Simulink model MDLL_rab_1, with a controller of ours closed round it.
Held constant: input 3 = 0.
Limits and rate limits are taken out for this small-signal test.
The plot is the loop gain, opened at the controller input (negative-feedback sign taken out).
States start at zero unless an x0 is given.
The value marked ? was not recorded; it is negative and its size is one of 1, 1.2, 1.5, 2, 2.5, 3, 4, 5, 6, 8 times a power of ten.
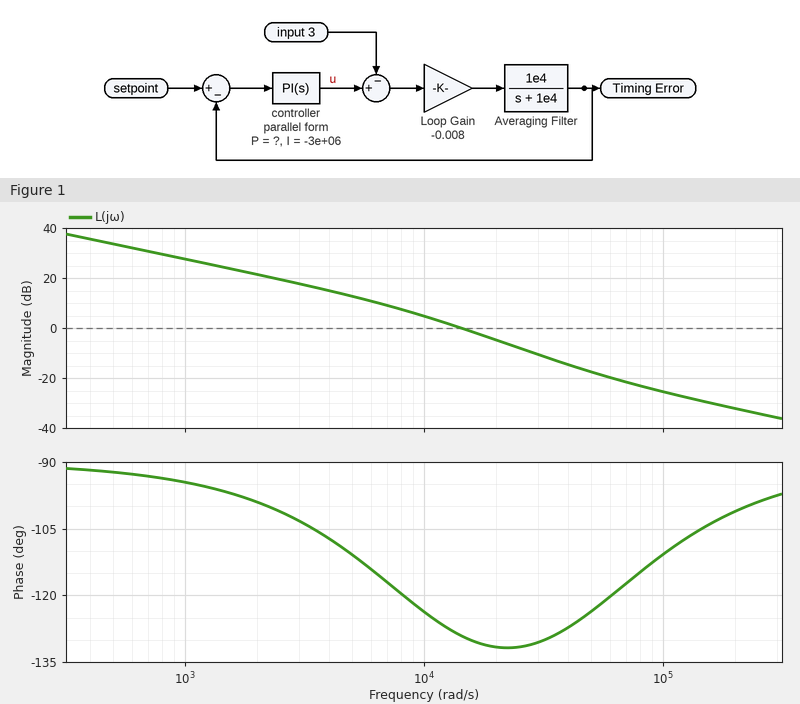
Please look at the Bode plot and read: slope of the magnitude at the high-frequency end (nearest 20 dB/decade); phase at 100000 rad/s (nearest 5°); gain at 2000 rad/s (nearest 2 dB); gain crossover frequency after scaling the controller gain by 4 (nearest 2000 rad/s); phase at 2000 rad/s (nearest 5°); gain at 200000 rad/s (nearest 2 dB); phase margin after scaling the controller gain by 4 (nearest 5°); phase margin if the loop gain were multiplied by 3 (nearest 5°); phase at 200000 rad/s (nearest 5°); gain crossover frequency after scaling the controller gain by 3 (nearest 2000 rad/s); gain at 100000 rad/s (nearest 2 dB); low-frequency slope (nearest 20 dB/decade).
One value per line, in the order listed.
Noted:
-20 dB/decade
-110°
22 dB
34000 rad/s
-100°
-32 dB
50°
50°
-100°
28000 rad/s
-26 dB
-20 dB/decade
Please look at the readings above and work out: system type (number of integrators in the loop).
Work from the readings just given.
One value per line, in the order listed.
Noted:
1
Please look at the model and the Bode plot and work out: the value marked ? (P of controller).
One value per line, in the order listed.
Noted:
-60
